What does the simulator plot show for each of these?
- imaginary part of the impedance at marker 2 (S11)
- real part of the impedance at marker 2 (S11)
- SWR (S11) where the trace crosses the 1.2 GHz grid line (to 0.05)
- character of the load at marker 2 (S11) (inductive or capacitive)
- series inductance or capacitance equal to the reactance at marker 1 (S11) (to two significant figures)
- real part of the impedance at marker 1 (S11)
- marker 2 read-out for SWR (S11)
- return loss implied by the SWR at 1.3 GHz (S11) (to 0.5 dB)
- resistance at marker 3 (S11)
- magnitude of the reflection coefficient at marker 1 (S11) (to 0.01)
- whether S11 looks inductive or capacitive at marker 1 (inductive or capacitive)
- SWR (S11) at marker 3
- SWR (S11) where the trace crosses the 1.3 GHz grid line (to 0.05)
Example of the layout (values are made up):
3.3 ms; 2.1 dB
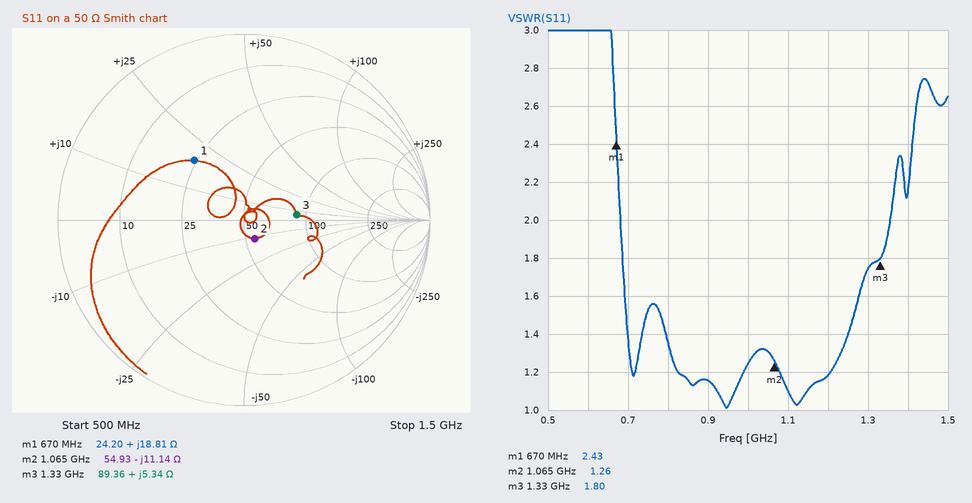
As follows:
-11.14 Ω; 54.93 Ω; 1.20; capacitive; 4.5 nH; 24.20 Ω; 1.26; 11.5 dB; 89.36 Ω; 0.42; inductive; 1.80; 1.75
